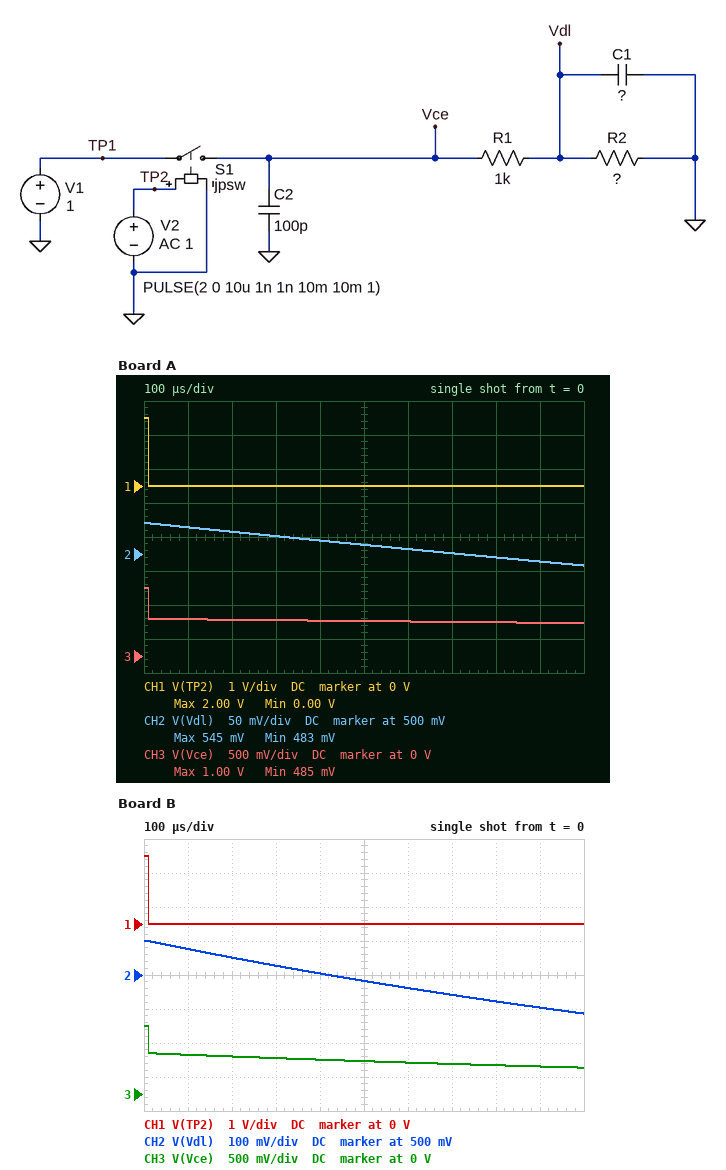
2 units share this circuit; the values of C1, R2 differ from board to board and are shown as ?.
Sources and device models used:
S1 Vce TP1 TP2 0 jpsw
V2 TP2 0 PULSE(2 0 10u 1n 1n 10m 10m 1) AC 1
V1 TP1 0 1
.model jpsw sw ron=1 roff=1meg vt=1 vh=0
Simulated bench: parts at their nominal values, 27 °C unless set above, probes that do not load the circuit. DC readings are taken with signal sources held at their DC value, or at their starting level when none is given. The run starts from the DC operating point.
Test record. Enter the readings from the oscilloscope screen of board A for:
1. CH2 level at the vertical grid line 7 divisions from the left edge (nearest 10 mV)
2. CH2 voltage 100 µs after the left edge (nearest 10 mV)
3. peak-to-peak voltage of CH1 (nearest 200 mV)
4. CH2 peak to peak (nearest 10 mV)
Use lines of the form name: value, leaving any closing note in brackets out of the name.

CH2 level at the vertical grid line 7 divisions from the left edge: 500 mV
CH2 voltage 100 µs after the left edge: 540 mV
peak-to-peak voltage of CH1: 2.0 V
CH2 peak to peak: 60 mV
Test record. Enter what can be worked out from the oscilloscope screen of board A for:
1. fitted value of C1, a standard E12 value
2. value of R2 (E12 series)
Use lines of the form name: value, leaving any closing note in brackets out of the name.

fitted value of C1, a standard E12 value: 6.8 µF
value of R2: 1.2 kΩ
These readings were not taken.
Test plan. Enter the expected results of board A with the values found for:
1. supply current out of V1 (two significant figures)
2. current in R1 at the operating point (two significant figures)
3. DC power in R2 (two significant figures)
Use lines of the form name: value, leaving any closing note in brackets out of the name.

supply current out of V1: 450 µA
current in R1 at the operating point: 450 µA
DC power in R2: 250 µW
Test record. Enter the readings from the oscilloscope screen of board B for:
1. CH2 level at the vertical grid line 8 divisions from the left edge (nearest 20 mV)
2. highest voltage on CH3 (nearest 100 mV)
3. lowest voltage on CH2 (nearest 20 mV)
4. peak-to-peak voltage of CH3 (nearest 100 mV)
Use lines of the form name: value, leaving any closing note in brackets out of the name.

CH2 level at the vertical grid line 8 divisions from the left edge: 420 mV
highest voltage on CH3: 1.0 V
lowest voltage on CH2: 380 mV
peak-to-peak voltage of CH3: 600 mV
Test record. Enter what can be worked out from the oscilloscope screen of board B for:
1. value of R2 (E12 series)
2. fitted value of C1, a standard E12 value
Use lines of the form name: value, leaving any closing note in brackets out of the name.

value of R2: 1.5 kΩ
fitted value of C1, a standard E12 value: 1.5 µF
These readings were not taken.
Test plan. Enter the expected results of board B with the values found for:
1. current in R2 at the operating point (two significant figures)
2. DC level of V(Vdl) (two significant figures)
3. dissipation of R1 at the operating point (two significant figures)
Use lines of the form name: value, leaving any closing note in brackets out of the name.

current in R2 at the operating point: 400 µA
DC level of V(Vdl): 600 mV
dissipation of R1 at the operating point: 160 µW
